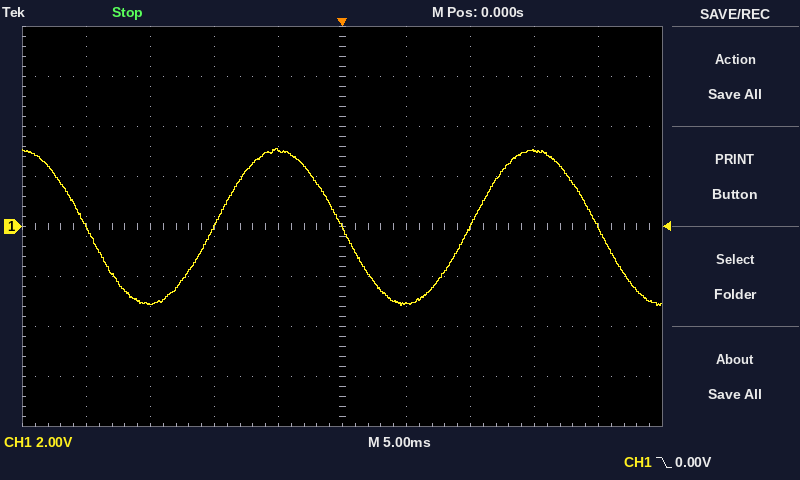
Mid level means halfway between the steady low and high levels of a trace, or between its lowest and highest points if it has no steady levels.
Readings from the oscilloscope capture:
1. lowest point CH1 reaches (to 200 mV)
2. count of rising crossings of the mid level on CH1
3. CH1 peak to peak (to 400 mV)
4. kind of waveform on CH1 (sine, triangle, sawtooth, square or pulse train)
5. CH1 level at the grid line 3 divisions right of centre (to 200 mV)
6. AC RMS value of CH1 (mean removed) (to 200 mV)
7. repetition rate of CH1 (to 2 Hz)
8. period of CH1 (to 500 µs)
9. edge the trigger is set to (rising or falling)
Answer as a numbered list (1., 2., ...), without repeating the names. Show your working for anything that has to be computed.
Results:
1. -3.2 V
2. 2
3. 6.4 V
4. sine
5. 3.0 V
6. 6.4 V / (2√2) ≈ 2.26 V, so 2.2 V to the nearest 200 mV
7. 1 / 20.0 ms ≈ 50 Hz
8. 20.0 ms
9. falling
